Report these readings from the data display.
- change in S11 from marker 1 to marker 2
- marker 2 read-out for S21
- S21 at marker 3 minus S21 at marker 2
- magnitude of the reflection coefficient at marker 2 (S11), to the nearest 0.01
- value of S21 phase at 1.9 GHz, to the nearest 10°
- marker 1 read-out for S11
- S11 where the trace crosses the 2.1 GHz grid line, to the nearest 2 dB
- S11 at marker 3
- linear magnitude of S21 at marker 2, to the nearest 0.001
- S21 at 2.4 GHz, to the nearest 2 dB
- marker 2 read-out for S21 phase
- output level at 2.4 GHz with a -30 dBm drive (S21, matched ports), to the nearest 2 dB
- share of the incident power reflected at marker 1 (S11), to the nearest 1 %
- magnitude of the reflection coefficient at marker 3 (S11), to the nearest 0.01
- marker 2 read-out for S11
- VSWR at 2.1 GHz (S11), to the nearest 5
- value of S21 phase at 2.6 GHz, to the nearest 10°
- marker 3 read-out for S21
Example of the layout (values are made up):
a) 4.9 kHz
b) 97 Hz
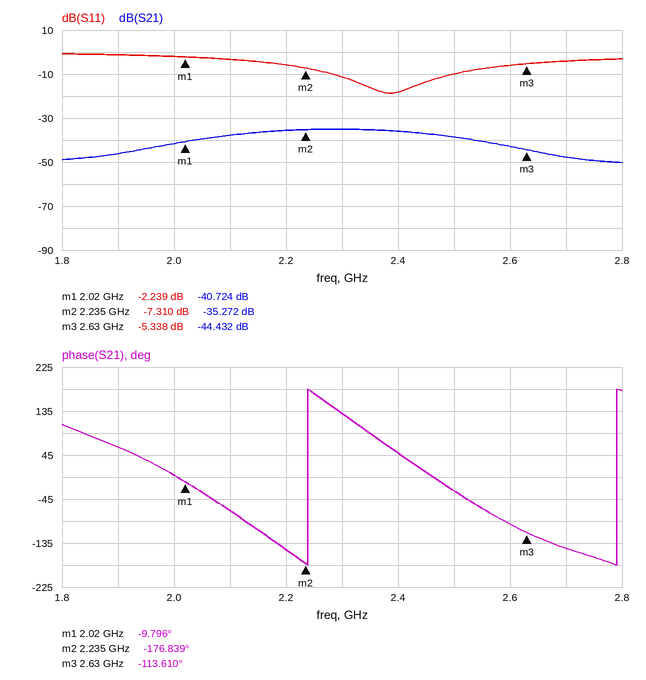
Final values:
a) -5.071 dB
b) -35.272 dB
c) -9.160 dB
d) 0.43
e) 60°
f) -2.239 dB
g) -4 dB
h) -5.338 dB
i) 0.017
j) -36 dB
k) -176.839°
l) -66 dBm
m) 60 %
n) 0.54
o) -7.310 dB
p) 5
q) -100°
r) -44.432 dB
